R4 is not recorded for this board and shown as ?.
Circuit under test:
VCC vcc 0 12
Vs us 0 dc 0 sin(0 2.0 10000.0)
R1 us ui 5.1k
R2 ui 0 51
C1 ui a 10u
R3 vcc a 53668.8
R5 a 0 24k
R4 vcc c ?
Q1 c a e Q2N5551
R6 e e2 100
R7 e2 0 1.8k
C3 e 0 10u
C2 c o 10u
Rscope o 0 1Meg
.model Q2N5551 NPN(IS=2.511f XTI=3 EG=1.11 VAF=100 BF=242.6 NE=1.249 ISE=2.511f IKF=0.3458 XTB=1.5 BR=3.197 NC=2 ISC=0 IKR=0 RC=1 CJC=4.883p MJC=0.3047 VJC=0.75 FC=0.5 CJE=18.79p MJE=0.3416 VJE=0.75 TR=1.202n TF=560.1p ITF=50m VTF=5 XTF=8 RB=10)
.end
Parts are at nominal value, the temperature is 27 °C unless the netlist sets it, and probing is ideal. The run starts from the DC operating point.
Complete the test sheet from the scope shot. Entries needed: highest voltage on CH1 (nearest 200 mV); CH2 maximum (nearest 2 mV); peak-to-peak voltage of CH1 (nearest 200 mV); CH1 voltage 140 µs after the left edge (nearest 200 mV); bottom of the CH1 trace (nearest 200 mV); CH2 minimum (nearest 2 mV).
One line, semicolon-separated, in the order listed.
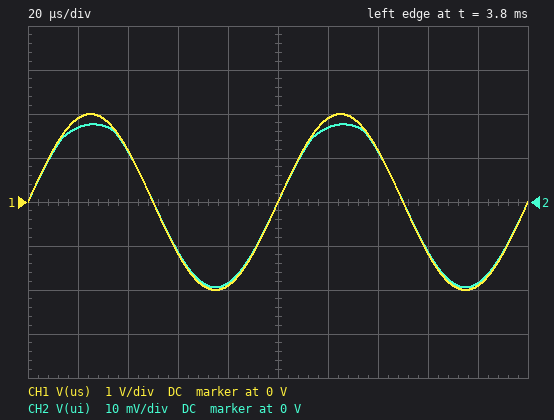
2.0 V; 18 mV; 4.0 V; 1.2 V; -2.0 V; -20 mV
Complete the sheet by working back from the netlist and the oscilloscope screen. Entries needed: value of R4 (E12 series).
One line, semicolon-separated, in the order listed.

3.9 kΩ
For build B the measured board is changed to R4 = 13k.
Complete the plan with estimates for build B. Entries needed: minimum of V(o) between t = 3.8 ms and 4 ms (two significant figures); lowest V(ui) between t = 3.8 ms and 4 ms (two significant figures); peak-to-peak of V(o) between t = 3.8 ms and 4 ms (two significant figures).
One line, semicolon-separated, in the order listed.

-23 mV; -16 mV; 2.2 V
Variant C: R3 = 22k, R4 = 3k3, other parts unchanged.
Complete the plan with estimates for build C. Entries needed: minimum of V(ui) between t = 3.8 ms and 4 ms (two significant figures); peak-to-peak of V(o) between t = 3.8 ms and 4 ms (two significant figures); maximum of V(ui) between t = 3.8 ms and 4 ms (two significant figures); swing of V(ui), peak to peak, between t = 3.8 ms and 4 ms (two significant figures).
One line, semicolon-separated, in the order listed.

-16 mV; 2.0 V; 7.7 mV; 23 mV
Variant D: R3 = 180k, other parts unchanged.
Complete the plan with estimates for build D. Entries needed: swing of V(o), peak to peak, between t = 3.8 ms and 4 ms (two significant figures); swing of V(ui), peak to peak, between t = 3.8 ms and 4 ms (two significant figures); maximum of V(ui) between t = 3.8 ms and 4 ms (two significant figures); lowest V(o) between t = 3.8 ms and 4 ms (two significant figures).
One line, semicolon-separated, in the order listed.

2.0 V; 39 mV; 20 mV; -1.2 V
